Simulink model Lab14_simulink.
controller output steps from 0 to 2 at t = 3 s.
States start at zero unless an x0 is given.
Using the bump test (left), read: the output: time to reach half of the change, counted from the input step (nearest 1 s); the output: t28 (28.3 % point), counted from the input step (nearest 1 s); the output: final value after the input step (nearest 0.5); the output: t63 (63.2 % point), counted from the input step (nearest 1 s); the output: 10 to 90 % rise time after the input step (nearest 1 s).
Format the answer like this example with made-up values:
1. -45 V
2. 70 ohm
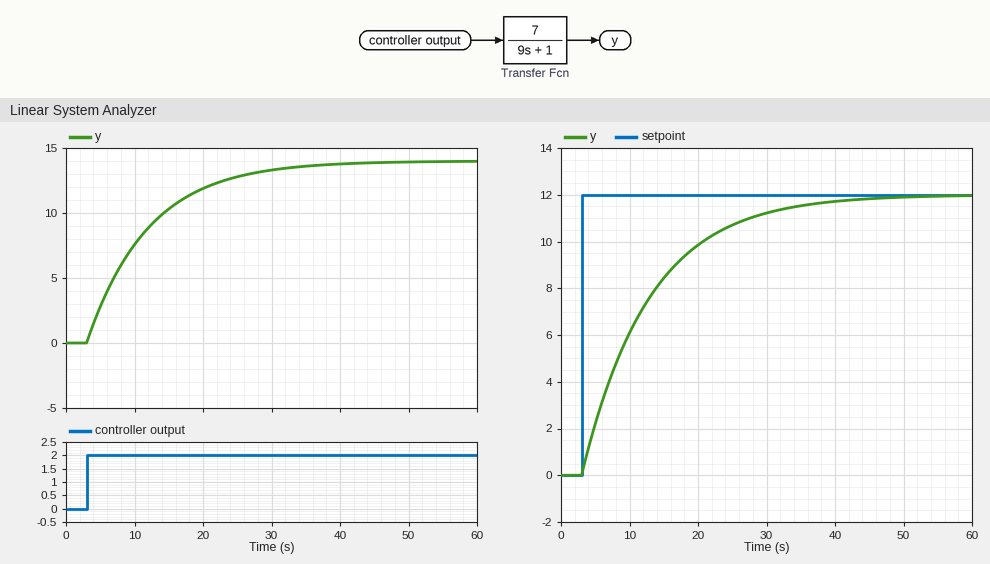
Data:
1. 6 s
2. 3 s
3. 14.0
4. 9 s
5. 20 s
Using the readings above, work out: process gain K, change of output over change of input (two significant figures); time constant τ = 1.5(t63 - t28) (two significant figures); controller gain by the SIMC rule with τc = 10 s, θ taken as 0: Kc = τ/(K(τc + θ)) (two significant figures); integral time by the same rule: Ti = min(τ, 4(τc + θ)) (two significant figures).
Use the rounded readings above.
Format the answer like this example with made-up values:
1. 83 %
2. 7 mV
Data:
1. 7.0
2. 9.0 s
3. 0.13
4. 9.0 s
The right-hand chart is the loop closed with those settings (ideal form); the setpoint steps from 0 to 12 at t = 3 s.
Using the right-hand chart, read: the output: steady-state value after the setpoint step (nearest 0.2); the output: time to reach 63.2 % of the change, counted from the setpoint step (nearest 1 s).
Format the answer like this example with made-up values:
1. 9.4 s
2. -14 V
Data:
1. 12.0
2. 10 s
